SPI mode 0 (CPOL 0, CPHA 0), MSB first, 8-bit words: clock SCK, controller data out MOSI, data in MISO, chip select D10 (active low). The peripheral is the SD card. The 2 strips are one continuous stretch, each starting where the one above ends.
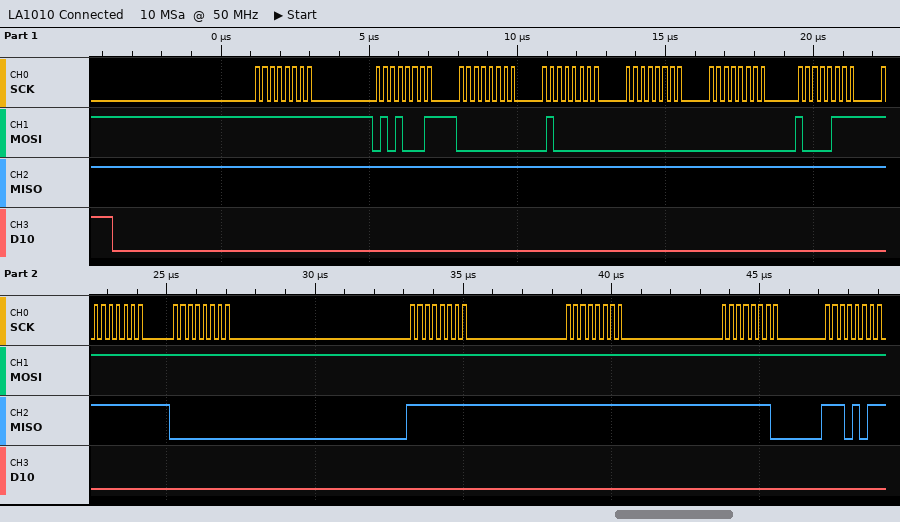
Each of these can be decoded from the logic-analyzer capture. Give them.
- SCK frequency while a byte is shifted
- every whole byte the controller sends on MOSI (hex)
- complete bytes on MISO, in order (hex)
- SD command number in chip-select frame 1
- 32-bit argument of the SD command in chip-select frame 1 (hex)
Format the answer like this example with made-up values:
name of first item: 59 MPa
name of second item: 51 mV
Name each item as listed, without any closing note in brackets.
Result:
SCK frequency while a byte is shifted: 4 MHz
every whole byte the controller sends on MOSI: FF 51 00 40 00 00 87 FF FF FF FF FF FF
complete bytes on MISO, in order: FF FF FF FF FF FF FF FF 00 FF FF FE EB
SD command number in chip-select frame 1: CMD17
32-bit argument of the SD command in chip-select frame 1: 0x00400000
